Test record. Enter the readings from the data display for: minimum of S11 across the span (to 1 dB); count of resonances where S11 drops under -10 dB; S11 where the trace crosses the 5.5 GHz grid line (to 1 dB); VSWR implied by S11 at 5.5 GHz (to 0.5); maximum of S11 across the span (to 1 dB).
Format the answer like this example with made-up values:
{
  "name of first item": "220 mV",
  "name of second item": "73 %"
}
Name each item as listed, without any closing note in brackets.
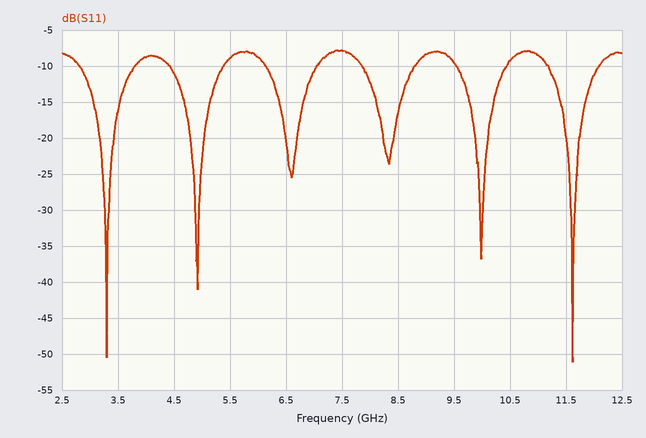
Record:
{
  "minimum of S11 across the span": "-51 dB",
  "count of resonances where S11 drops under -10 dB": "6",
  "S11 where the trace crosses the 5.5 GHz grid line": "-9 dB",
  "VSWR implied by S11 at 5.5 GHz": "2.0",
  "maximum of S11 across the span": "-8 dB"
}
